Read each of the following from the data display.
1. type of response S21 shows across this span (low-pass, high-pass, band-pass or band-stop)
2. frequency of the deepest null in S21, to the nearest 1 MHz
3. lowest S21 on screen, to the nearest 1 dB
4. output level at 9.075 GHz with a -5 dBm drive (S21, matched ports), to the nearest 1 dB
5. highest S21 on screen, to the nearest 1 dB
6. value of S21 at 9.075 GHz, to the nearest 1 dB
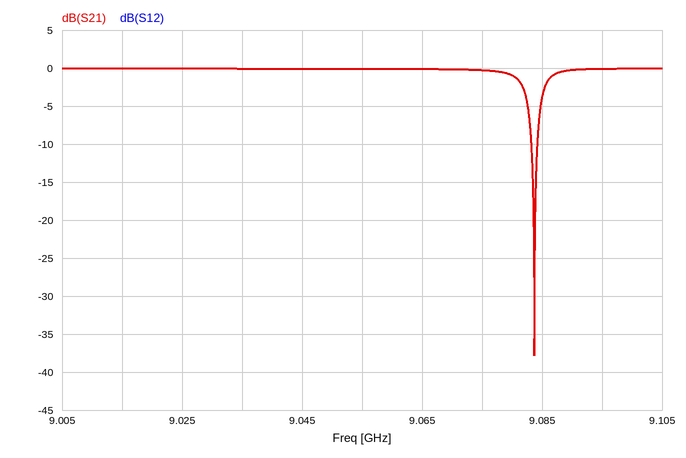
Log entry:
band-stop
9.084 GHz
-38 dB
-5 dBm
0 dB
0 dB
